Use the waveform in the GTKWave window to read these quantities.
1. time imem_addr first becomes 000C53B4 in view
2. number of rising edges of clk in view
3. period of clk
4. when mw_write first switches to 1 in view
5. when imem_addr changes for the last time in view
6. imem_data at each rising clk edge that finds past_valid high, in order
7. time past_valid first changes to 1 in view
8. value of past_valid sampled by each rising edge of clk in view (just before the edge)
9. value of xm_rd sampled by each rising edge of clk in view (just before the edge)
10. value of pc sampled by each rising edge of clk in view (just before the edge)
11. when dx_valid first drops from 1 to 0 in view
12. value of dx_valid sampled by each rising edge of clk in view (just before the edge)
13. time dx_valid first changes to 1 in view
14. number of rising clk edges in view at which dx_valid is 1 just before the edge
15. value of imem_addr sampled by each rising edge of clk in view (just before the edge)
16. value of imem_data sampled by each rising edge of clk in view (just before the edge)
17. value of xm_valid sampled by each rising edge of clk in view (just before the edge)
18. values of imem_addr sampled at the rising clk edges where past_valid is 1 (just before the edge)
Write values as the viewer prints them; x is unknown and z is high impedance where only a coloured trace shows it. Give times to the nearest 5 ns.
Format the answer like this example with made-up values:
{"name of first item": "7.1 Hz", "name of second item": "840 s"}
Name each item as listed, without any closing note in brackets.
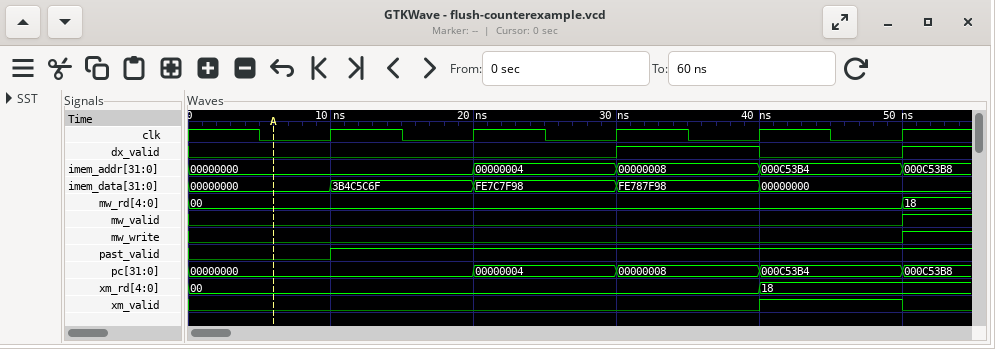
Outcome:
{"time imem_addr first becomes 000C53B4 in view": "40 ns", "number of rising edges of clk in view": "5", "period of clk": "10 ns", "when mw_write first switches to 1 in view": "50 ns", "when imem_addr changes for the last time in view": "50 ns", "imem_data at each rising clk edge that finds past_valid high, in order": "3B4C5C6F, FE7C7F98, FE787F98, 00000000", "time past_valid first changes to 1 in view": "10 ns", "value of past_valid sampled by each rising edge of clk in view": "0 1 1 1 1", "value of xm_rd sampled by each rising edge of clk in view": "00, 00, 00, 00, 18", "value of pc sampled by each rising edge of clk in view": "00000000, 00000000, 00000004, 00000008, 000C53B4", "when dx_valid first drops from 1 to 0 in view": "40 ns", "value of dx_valid sampled by each rising edge of clk in view": "0 0 0 1 0", "time dx_valid first changes to 1 in view": "30 ns", "number of rising clk edges in view at which dx_valid is 1 just before the edge": "1", "value of imem_addr sampled by each rising edge of clk in view": "00000000, 00000000, 00000004, 00000008, 000C53B4", "value of imem_data sampled by each rising edge of clk in view": "00000000, 3B4C5C6F, FE7C7F98, FE787F98, 00000000", "value of xm_valid sampled by each rising edge of clk in view": "0 0 0 0 1", "values of imem_addr sampled at the rising clk edges where past_valid is 1": "00000000, 00000004, 00000008, 000C53B4"}
